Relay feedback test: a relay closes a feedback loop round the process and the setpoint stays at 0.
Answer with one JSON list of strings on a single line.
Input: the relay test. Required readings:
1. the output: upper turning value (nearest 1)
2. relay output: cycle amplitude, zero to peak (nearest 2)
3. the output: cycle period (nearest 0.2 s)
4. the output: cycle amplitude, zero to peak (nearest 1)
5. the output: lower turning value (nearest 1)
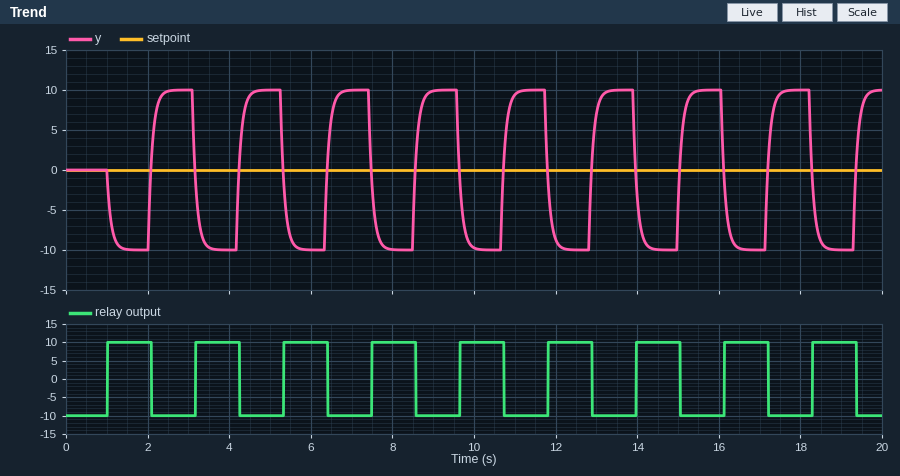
["10", "10", "2.2 s", "10", "-10"]
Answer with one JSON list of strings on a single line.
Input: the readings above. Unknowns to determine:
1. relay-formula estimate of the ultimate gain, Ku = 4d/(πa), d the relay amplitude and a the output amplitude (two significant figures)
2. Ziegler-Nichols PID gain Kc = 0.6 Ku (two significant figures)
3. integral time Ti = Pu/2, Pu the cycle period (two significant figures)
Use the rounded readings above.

["1.3", "0.78", "1.1 s"]
